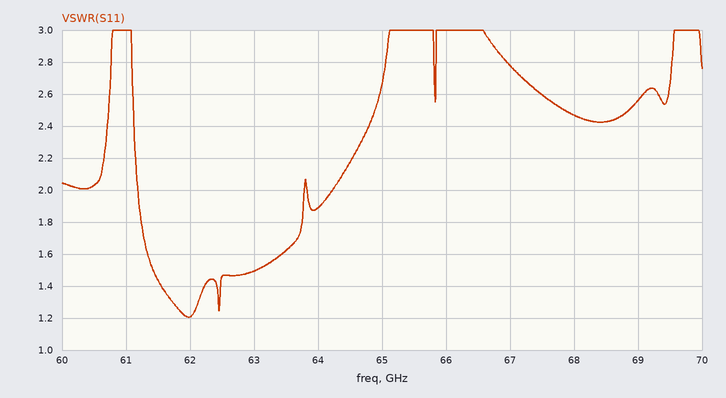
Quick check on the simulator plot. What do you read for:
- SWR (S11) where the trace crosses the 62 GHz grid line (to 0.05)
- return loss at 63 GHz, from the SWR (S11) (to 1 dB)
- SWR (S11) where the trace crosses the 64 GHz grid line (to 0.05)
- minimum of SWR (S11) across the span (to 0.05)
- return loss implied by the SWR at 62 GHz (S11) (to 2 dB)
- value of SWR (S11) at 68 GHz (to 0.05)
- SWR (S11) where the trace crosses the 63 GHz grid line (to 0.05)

1.20
14 dB
1.90
1.20
20 dB
2.45
1.50
